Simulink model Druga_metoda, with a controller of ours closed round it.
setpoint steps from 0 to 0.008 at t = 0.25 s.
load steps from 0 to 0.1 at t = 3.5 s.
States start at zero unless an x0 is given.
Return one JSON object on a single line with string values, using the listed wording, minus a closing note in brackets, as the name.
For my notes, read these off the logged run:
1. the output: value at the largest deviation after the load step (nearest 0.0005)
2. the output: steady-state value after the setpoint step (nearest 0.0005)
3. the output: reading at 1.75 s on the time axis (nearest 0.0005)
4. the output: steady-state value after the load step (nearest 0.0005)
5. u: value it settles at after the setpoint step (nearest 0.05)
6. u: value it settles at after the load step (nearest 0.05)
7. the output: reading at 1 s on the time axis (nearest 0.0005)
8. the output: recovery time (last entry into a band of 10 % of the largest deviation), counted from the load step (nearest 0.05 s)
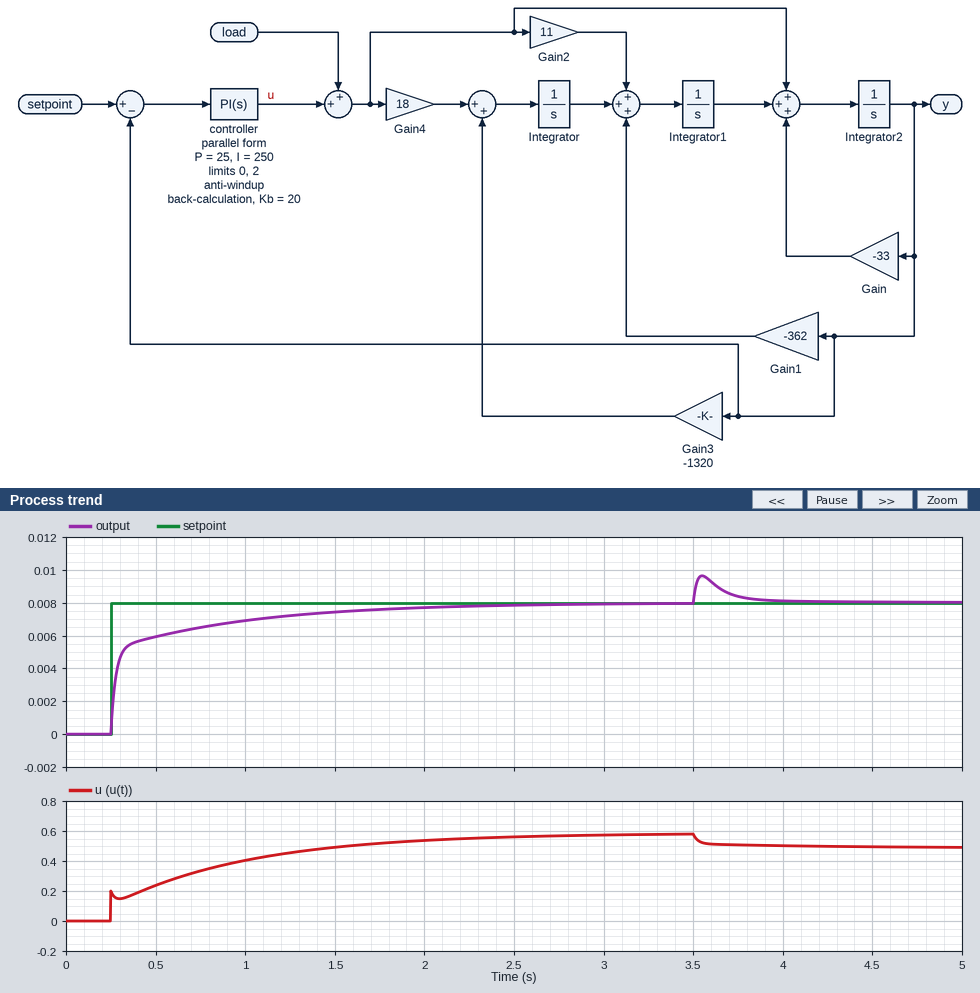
{"the output: value at the largest deviation after the load step": "0.0095", "the output: steady-state value after the setpoint step": "0.0080", "the output: reading at 1.75 s on the time axis": "0.0075", "the output: steady-state value after the load step": "0.0080", "u: value it settles at after the setpoint step": "0.60", "u: value it settles at after the load step": "0.50", "the output: reading at 1 s on the time axis": "0.0070", "the output: recovery time (last entry into a band of 10 % of the largest deviation), counted from the load step": "0.40 s"}
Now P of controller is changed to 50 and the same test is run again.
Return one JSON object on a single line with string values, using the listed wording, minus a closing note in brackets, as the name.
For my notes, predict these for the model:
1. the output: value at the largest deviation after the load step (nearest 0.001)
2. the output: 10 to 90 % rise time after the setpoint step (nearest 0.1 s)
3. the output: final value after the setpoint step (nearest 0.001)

{"the output: value at the largest deviation after the load step": "0.009", "the output: 10 to 90 % rise time after the setpoint step": "1.1 s", "the output: final value after the setpoint step": "0.008"}
